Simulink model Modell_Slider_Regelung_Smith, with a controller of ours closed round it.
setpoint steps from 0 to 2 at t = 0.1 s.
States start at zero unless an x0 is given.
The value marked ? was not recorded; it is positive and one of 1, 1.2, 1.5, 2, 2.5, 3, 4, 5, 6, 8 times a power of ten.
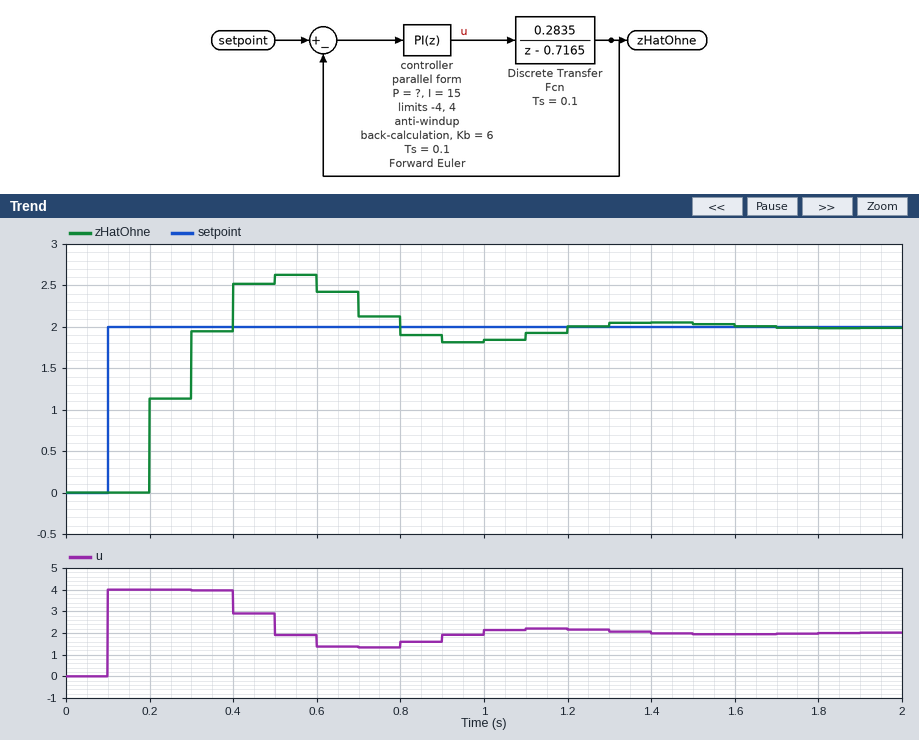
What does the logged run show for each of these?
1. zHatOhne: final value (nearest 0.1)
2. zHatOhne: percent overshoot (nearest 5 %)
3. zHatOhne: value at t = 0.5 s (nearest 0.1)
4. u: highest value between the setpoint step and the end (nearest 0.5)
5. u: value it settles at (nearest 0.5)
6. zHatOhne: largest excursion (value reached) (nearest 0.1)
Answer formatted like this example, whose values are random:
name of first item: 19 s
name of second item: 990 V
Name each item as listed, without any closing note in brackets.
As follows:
zHatOhne: final value: 2.0
zHatOhne: percent overshoot: 30 %
zHatOhne: value at t = 0.5 s: 2.6
u: highest value between the setpoint step and the end: 4.0
u: value it settles at: 2.0
zHatOhne: largest excursion (value reached): 2.6
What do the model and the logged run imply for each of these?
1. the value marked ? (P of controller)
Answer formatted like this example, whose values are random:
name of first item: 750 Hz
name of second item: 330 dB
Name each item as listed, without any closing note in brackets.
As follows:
the value marked ?: 2
